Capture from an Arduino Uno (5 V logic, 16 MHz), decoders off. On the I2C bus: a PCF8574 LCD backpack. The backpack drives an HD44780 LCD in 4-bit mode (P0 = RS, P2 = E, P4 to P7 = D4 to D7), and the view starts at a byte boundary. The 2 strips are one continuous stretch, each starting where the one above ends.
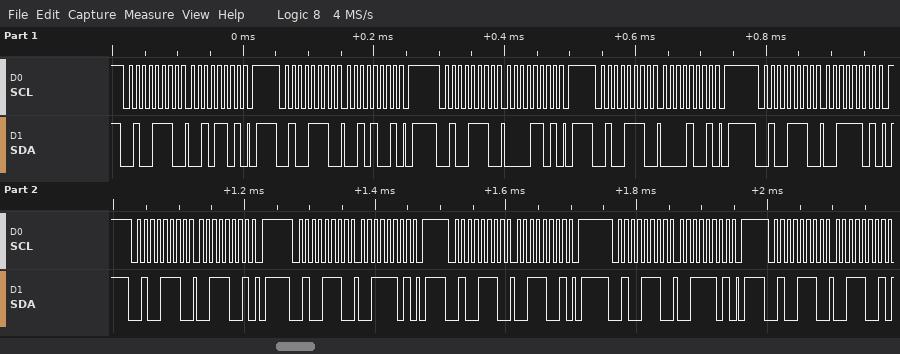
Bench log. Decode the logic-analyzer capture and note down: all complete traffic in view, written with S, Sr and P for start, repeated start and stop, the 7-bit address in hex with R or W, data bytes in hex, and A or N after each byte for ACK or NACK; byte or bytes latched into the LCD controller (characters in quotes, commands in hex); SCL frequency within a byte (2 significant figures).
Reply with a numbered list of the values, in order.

1. S 27W A 2D A P S 27W A 29 A P S 27W A 0D A P S 27W A 09 A P S 27W A 3D A P S 27W A 39 A P S 27W A 3D A P S 27W A 39 A P S 27W A 3D A P S 27W A 39 A
2. ' ' '3'
3. 100 kHz
